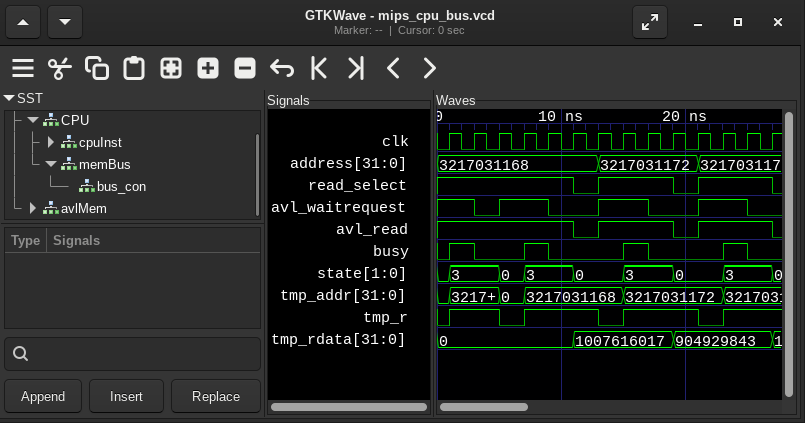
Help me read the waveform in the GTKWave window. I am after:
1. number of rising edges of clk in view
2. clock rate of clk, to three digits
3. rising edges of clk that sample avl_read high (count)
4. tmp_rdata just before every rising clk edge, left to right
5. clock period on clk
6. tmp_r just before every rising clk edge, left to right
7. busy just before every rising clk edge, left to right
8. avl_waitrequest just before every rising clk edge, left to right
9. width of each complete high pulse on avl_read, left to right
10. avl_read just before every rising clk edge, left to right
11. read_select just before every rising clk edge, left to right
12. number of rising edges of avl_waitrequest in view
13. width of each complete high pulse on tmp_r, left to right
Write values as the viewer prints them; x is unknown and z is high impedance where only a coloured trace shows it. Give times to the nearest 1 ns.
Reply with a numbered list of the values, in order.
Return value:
1. 14
2. 500 MHz
3. 12
4. 0, 0, 0, 0, 0, 0, 1007616017, 1007616017, 1007616017, 1007616017, 904929843, 904929843, 904929843, 904929843
5. 2 ns
6. 0 1 1 0 1 1 1 0 1 1 1 0 1 1
7. 0 1 0 0 1 0 0 0 1 0 0 0 1 0
8. 1 1 0 1 1 0 0 1 1 0 0 1 1 0
9. 6 ns, 6 ns
10. 1 1 1 1 1 1 0 1 1 1 0 1 1 1
11. 1 1 1 1 1 1 0 1 1 1 0 1 1 1
12. 3
13. 4 ns, 6 ns, 6 ns
